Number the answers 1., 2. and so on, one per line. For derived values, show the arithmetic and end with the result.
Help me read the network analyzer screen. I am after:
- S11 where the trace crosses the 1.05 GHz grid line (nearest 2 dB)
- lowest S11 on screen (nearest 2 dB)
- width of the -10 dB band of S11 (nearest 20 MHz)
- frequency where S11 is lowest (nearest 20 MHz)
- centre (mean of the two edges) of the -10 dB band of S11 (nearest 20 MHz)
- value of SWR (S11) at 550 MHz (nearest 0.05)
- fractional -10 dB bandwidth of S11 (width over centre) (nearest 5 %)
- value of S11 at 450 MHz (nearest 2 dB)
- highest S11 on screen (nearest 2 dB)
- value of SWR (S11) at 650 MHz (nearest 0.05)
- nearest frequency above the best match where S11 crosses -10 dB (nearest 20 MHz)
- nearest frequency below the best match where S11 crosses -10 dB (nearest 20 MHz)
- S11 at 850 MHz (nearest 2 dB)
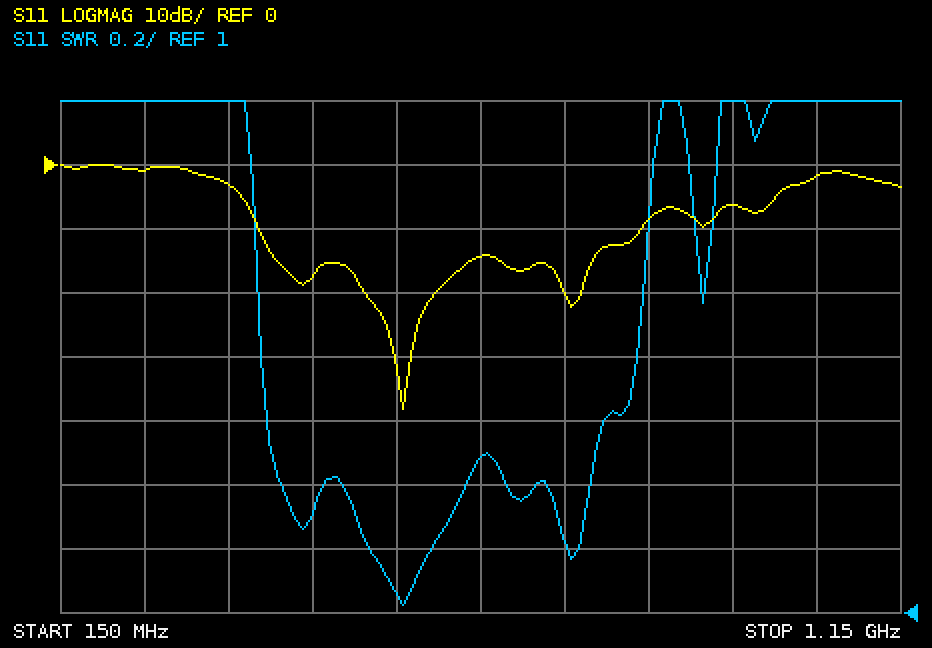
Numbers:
1. -2 dB
2. -38 dB
3. 840 MHz − 380 MHz = 460 MHz
4. 560 MHz
5. 620 MHz
6. 1.05
7. 460 MHz / 610 MHz ≈ 75 %
8. -18 dB
9. 0 dB
10. 1.50
11. 840 MHz
12. 380 MHz
13. -8 dB
